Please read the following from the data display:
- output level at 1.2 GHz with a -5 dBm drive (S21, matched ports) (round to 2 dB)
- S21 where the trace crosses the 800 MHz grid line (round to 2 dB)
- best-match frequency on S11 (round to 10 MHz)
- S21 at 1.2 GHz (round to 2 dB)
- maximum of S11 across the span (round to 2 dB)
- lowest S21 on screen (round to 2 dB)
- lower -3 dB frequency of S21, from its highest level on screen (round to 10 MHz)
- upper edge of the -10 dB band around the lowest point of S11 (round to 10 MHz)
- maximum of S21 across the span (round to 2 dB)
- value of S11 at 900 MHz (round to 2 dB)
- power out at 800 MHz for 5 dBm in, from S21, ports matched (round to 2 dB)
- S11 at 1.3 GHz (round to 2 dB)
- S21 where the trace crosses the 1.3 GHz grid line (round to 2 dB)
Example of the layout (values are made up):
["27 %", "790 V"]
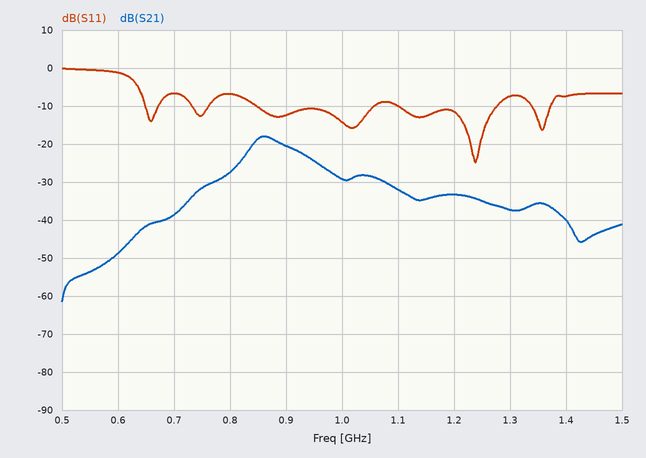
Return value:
["-38 dBm", "-28 dB", "1.24 GHz", "-34 dB", "0 dB", "-62 dB", "840 MHz", "1.28 GHz", "-18 dB", "-12 dB", "-22 dBm", "-8 dB", "-38 dB"]
